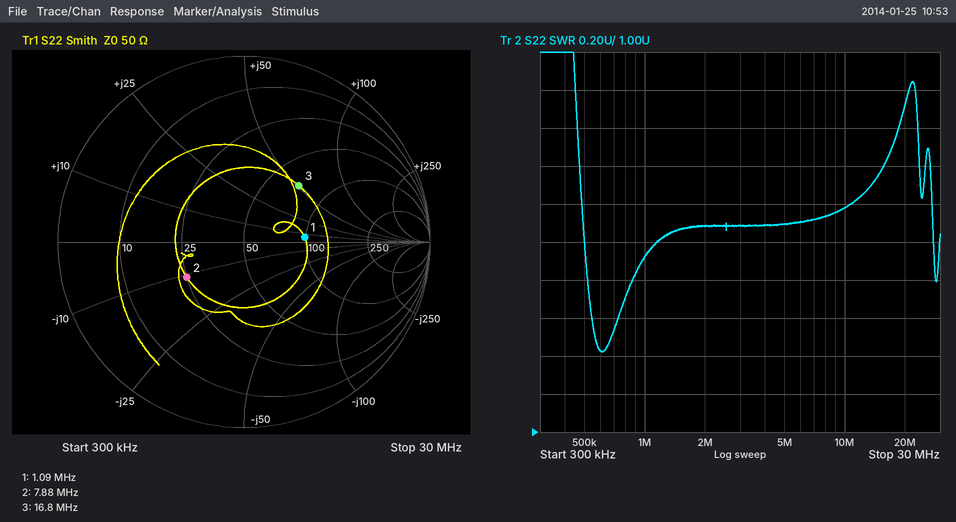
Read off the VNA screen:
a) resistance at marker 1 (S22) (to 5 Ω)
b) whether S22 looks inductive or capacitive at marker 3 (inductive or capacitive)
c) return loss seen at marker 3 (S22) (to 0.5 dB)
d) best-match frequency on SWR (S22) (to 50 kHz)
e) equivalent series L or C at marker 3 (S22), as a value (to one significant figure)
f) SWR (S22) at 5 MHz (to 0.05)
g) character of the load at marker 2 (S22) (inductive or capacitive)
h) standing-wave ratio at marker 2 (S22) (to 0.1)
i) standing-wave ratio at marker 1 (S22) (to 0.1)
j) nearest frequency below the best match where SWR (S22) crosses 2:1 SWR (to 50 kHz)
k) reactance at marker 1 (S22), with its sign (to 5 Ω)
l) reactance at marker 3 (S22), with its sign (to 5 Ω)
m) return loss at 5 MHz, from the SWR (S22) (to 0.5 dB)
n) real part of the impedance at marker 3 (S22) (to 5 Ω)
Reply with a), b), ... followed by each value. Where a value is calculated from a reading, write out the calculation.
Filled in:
a) 100 Ω
b) inductive
c) 7.5 dB
d) 600 kHz
e) L = 50 Ω/(2π × 16.8 MHz) ≈ 474 nH, so 500 nH to one significant figure
f) 2.10
g) capacitive
h) 2.1
i) 2.0
j) 500 kHz
k) +5 Ω
l) +50 Ω
m) −20 log10((2.1 − 1)/(2.1 + 1)) ≈ 9.0 dB
n) 70 Ω
